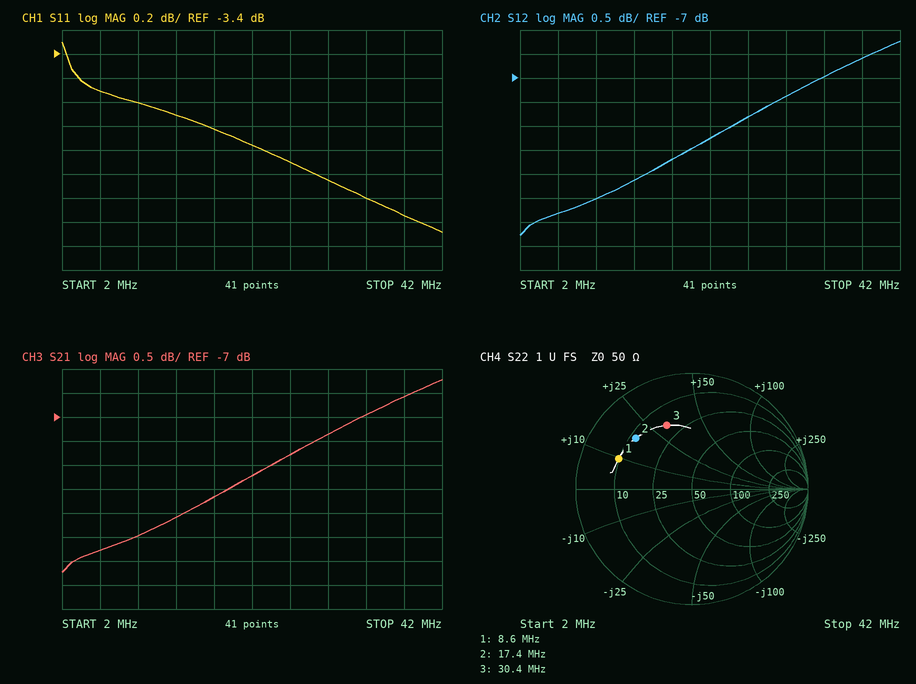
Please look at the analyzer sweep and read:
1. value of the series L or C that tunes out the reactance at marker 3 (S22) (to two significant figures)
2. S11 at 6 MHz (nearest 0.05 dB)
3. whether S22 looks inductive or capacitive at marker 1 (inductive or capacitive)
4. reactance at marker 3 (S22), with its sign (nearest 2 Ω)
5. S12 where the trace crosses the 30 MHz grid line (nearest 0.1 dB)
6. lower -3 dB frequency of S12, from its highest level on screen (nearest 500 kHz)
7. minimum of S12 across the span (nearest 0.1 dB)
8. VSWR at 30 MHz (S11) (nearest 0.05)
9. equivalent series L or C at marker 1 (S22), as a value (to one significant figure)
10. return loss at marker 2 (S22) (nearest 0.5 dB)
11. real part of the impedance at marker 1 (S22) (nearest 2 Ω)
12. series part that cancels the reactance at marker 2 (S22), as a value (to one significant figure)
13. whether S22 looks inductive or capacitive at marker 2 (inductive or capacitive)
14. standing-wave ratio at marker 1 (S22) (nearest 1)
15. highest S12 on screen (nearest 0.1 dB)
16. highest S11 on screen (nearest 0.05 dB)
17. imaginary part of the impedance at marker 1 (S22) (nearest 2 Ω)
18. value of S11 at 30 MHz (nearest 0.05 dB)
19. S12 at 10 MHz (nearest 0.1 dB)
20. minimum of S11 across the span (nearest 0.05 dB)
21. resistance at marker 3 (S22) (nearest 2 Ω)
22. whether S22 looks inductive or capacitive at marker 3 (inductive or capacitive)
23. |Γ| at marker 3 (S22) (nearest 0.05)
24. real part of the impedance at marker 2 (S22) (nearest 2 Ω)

170 pF
-3.70 dB
inductive
+30 Ω
-7.4 dB
13.0 MHz
-10.3 dB
4.00
200 nH
3.5 dB
10 Ω
500 pF
inductive
5
-6.2 dB
-3.30 dB
+10 Ω
-4.45 dB
-9.5 dB
-4.90 dB
18 Ω
inductive
0.60
12 Ω
